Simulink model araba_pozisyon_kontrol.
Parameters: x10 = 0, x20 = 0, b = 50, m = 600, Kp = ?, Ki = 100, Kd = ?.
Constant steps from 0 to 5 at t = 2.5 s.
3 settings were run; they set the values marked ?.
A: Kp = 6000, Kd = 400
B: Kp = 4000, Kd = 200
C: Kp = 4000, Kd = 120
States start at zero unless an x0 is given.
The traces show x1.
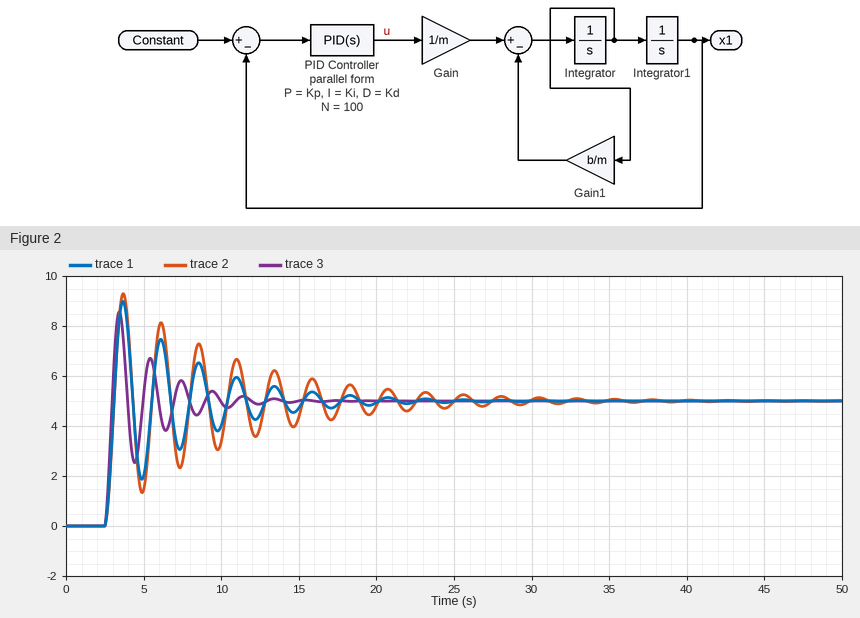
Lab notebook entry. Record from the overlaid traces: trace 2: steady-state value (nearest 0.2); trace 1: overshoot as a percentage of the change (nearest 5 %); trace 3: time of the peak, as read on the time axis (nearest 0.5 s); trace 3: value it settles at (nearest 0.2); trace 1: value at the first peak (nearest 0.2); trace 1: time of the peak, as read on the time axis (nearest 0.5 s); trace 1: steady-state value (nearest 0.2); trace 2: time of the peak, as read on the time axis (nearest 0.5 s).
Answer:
5.0
80 %
3.5 s
5.0
9.0
3.5 s
5.0
3.5 s
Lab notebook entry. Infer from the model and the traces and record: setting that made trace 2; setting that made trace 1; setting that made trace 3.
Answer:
C
B
A
